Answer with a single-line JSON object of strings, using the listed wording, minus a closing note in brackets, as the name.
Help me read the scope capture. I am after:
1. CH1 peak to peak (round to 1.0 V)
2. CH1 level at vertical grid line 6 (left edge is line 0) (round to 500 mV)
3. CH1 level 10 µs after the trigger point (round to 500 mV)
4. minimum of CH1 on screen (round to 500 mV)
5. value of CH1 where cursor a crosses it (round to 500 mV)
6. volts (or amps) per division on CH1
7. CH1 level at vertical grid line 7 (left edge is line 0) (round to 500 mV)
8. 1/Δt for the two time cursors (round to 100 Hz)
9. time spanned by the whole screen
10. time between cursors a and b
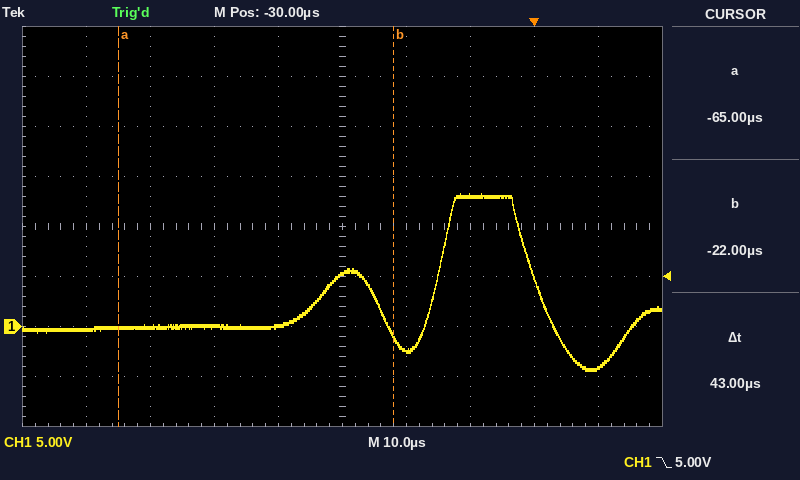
{"CH1 peak to peak": "18.0 V", "CH1 level at vertical grid line 6 (left edge is line 0)": "-2.5 V", "CH1 level 10 µs after the trigger point": "-4.0 V", "minimum of CH1 on screen": "-4.5 V", "value of CH1 where cursor a crosses it": "0.0 V", "volts (or amps) per division on CH1": "5 V", "CH1 level at vertical grid line 7 (left edge is line 0)": "13.0 V", "1/Δt for the two time cursors": "23.3 kHz", "time spanned by the whole screen": "100 µs", "time between cursors a and b": "43 µs"}
